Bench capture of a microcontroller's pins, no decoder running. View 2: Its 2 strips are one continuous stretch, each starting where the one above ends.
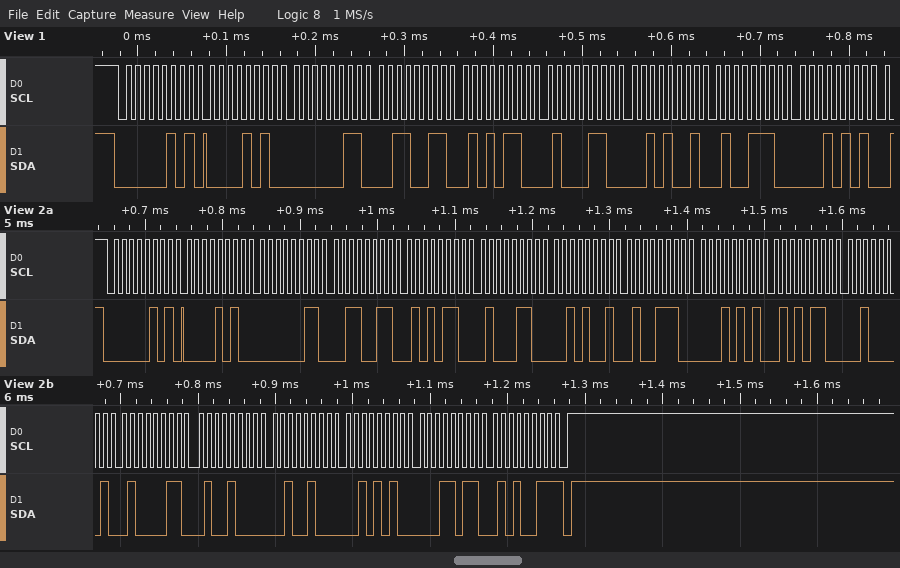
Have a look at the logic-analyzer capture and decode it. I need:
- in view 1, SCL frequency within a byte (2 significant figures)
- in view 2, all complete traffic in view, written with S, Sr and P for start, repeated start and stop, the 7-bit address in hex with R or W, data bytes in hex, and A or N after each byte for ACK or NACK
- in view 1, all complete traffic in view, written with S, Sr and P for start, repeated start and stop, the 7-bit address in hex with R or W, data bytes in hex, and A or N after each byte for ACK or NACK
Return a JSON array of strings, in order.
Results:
["100 kHz", "S 02R A 0A A 03 A 33 A 56 A 46 A 29 A 4E A 15 A 56 A 21 A 43 A 48 A 24 A 2A A 1B A 53 N P", "S 02R A 0A A 03 A 33 A 56 A 46 A 29 A 4E A 15 A"]
